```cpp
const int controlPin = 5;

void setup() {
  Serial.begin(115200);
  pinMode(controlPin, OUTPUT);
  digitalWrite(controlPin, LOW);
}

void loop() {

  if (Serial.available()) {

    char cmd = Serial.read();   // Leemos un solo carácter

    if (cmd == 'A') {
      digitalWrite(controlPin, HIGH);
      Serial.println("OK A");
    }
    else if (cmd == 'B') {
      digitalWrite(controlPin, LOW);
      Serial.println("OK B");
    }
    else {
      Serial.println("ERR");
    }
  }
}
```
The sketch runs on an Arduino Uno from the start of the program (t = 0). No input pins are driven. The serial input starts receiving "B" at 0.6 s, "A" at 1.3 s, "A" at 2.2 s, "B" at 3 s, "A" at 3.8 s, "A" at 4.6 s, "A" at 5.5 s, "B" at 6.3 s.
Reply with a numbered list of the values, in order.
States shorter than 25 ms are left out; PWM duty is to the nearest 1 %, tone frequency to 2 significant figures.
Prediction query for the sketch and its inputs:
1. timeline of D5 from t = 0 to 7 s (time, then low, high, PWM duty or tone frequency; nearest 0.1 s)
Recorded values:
1. 0 s low; 1.3 s high; 3 s low; 3.8 s high; 6.3 s low
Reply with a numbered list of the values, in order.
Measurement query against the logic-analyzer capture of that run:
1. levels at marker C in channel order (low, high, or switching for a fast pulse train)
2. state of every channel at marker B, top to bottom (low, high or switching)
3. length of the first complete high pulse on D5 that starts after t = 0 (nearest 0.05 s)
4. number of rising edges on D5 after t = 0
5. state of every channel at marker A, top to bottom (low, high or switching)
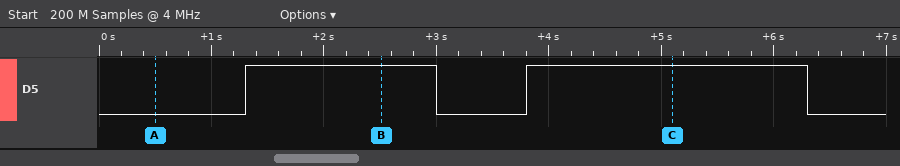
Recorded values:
1. D5 high
2. D5 high
3. 1.70 s
4. 2
5. D5 low
